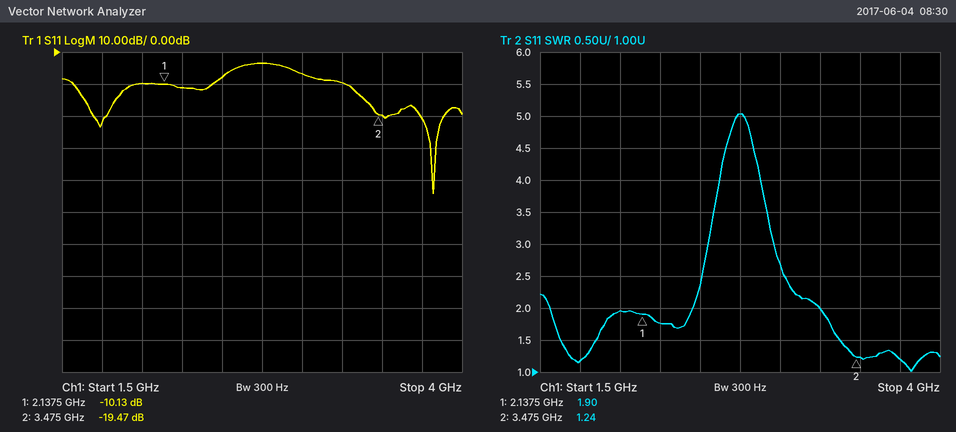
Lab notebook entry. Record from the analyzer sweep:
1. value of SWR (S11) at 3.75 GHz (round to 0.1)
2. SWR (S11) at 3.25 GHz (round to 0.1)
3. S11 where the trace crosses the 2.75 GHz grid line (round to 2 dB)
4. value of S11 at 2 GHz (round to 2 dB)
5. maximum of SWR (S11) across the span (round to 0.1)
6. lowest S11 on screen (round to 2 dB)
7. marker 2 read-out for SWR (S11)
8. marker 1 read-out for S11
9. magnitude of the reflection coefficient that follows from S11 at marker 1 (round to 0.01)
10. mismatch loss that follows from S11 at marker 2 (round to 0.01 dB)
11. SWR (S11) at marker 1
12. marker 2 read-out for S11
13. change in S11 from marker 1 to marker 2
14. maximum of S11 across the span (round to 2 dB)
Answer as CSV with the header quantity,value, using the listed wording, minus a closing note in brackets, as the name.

quantity,value
value of SWR (S11) at 3.75 GHz,1.2
SWR (S11) at 3.25 GHz,2.0
S11 where the trace crosses the 2.75 GHz grid line,-4 dB
value of S11 at 2 GHz,-10 dB
maximum of SWR (S11) across the span,5.0
lowest S11 on screen,-44 dB
marker 2 read-out for SWR,1.24
marker 1 read-out for S11,-10.13 dB
magnitude of the reflection coefficient that follows from S11 at marker 1,0.31
mismatch loss that follows from S11 at marker 2,0.05 dB
SWR (S11) at marker 1,1.90
marker 2 read-out for S11,-19.47 dB
change in S11 from marker 1 to marker 2,-9.34 dB
maximum of S11 across the span,-4 dB
